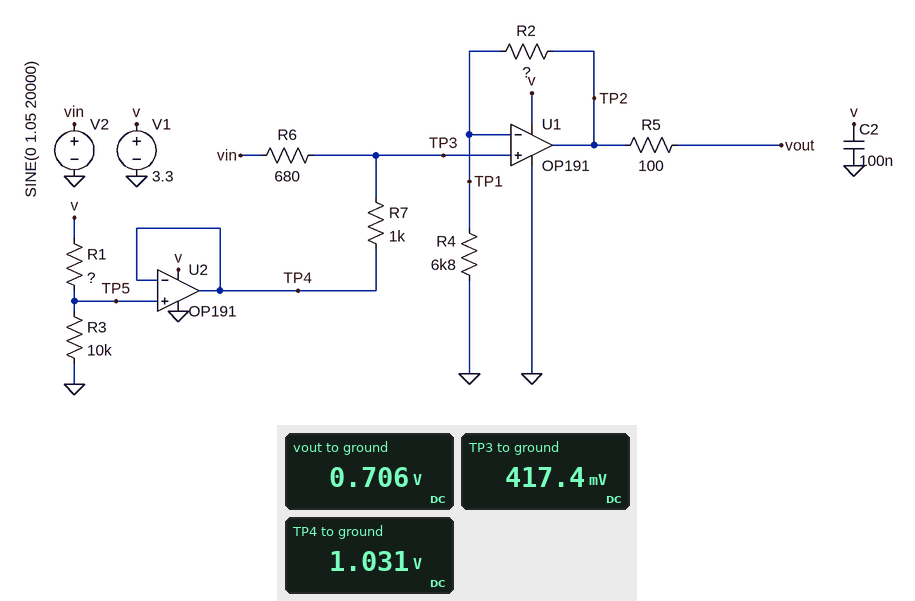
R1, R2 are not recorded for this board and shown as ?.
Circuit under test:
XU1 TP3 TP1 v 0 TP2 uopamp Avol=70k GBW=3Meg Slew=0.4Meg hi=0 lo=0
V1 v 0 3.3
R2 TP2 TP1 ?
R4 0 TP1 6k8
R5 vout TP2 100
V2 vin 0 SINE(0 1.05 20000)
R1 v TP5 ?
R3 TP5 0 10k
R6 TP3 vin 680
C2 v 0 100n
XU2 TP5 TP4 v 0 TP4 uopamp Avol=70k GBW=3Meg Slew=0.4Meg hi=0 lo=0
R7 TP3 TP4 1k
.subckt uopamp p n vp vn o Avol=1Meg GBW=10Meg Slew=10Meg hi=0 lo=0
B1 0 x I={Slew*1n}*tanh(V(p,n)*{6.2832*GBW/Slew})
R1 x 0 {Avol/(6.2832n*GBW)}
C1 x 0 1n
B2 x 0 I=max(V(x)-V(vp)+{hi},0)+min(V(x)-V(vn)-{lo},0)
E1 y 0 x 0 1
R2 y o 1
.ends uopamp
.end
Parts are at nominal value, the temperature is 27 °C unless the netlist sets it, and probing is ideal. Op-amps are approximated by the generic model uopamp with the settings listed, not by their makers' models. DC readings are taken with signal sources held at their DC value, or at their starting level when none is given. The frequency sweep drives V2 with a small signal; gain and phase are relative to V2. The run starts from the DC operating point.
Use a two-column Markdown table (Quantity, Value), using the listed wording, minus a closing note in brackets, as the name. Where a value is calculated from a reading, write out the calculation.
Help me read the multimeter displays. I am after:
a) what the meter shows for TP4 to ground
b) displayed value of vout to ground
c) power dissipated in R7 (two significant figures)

| Quantity | Value |
|---|---|
| what the meter shows for TP4 to ground | 1.031 V |
| displayed value of vout to ground | 0.706 V |
| power dissipated in R7 | (1.031 V - 417.4 mV)^2 / 1 kΩ = 380 µW |
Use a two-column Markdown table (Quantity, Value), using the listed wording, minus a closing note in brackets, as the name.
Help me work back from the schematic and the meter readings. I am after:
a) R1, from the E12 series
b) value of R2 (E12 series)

| Quantity | Value |
|---|---|
| R1, from the E12 series | 22 kΩ |
| value of R2 | 4.7 kΩ |
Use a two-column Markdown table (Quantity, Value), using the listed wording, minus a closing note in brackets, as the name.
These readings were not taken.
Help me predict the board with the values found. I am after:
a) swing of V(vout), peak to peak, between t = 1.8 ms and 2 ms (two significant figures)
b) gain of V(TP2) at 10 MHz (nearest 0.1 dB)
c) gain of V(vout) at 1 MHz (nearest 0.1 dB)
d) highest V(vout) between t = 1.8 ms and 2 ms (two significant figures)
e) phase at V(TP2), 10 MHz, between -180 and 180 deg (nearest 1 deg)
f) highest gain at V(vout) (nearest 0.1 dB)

| Quantity | Value |
|---|---|
| swing of V(vout), peak to peak, between t = 1.8 ms and 2 ms | 1.8 V |
| gain of V(TP2) at 10 MHz | -15.1 dB |
| gain of V(vout) at 1 MHz | -1.1 dB |
| highest V(vout) between t = 1.8 ms and 2 ms | 1.8 V |
| phase at V(TP2), 10 MHz, between -180 and 180 deg | -80 deg |
| highest gain at V(vout) | 0.1 dB |
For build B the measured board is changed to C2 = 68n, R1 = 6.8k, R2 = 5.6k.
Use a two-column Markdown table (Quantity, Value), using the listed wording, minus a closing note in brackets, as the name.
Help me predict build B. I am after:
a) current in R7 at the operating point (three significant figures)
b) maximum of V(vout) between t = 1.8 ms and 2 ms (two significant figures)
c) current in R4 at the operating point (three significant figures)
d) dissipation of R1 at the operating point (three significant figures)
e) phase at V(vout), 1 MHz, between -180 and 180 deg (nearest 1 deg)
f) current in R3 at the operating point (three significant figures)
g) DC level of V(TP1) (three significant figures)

| Quantity | Value |
|---|---|
| current in R7 at the operating point | 1.17 mA |
| maximum of V(vout) between t = 1.8 ms and 2 ms | 2.6 V |
| current in R4 at the operating point | 117 µA |
| dissipation of R1 at the operating point | 262 µW |
| phase at V(vout), 1 MHz, between -180 and 180 deg | -31 deg |
| current in R3 at the operating point | 196 µA |
| DC level of V(TP1) | 795 mV |
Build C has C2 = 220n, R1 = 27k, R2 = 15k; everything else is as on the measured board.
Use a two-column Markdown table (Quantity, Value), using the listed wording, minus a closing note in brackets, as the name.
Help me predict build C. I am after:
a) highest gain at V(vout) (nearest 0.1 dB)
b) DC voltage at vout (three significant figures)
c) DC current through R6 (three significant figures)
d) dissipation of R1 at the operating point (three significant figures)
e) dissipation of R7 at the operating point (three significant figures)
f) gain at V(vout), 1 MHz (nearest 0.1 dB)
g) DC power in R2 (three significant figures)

| Quantity | Value |
|---|---|
| highest gain at V(vout) | 5.6 dB |
| DC voltage at vout | 1.16 V |
| DC current through R6 | 531 µA |
| dissipation of R1 at the operating point | 215 µW |
| dissipation of R7 at the operating point | 282 µW |
| gain at V(vout), 1 MHz | 2.3 dB |
| DC power in R2 | 42.3 µW |
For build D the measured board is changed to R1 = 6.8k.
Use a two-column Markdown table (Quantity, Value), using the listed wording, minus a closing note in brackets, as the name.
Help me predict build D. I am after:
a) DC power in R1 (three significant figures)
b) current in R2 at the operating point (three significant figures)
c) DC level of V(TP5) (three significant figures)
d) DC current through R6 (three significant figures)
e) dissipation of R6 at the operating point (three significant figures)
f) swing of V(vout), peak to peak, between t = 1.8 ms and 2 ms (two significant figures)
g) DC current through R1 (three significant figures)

| Quantity | Value |
|---|---|
| DC power in R1 | 262 µW |
| current in R2 at the operating point | 117 µA |
| DC level of V(TP5) | 1.96 V |
| DC current through R6 | 1.17 mA |
| dissipation of R6 at the operating point | 930 µW |
| swing of V(vout), peak to peak, between t = 1.8 ms and 2 ms | 2.1 V |
| DC current through R1 | 196 µA |
